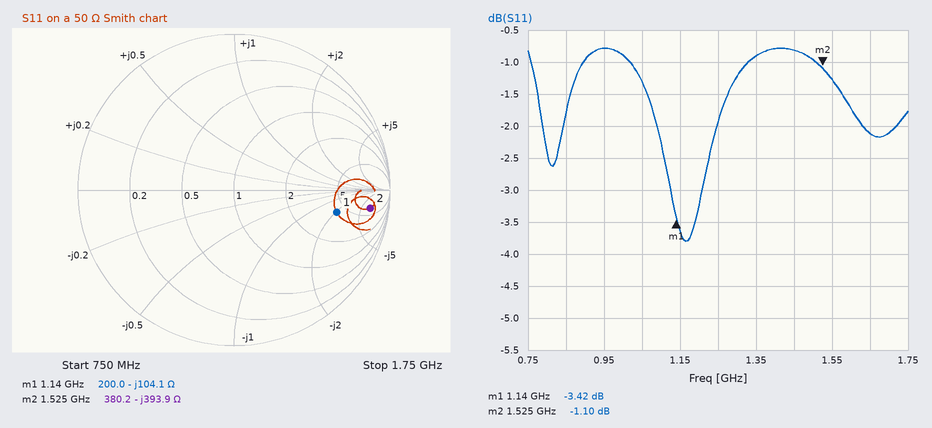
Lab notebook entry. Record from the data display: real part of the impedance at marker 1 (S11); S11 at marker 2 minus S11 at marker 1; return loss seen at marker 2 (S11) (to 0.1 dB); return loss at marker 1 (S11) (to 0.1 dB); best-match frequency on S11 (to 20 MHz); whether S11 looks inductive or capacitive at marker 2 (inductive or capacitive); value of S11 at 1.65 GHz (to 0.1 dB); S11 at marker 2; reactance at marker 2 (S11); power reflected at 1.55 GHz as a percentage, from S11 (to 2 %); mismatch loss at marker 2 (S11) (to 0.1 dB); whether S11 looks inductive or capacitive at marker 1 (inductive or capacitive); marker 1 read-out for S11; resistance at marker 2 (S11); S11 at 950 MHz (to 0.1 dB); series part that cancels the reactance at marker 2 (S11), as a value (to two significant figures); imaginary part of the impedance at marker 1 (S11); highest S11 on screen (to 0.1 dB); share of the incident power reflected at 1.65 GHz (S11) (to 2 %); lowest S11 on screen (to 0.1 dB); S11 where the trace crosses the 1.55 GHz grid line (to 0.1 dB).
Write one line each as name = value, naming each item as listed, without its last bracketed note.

real part of the impedance at marker 1 = 200.0 Ω
S11 at marker 2 minus S11 at marker 1 = 2.32 dB
return loss seen at marker 2 (S11) = 1.1 dB
return loss at marker 1 (S11) = 3.4 dB
best-match frequency on S11 = 1.16 GHz
whether S11 looks inductive or capacitive at marker 2 = capacitive
value of S11 at 1.65 GHz = -2.1 dB
S11 at marker 2 = -1.10 dB
reactance at marker 2 = -393.9 Ω
power reflected at 1.55 GHz as a percentage, from S11 = 74 %
mismatch loss at marker 2 (S11) = 6.5 dB
whether S11 looks inductive or capacitive at marker 1 = capacitive
marker 1 read-out for S11 = -3.42 dB
resistance at marker 2 = 380.2 Ω
S11 at 950 MHz = -0.8 dB
series part that cancels the reactance at marker 2 (S11), as a value = 41 nH
imaginary part of the impedance at marker 1 = -104.1 Ω
highest S11 on screen = -0.8 dB
share of the incident power reflected at 1.65 GHz (S11) = 62 %
lowest S11 on screen = -3.8 dB
S11 where the trace crosses the 1.55 GHz grid line = -1.3 dB
